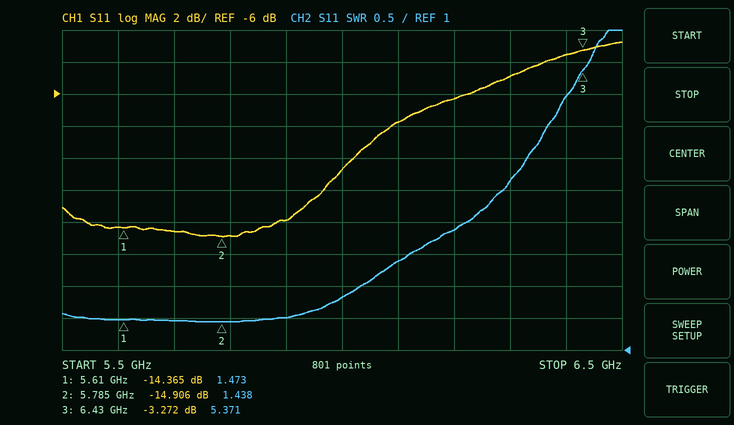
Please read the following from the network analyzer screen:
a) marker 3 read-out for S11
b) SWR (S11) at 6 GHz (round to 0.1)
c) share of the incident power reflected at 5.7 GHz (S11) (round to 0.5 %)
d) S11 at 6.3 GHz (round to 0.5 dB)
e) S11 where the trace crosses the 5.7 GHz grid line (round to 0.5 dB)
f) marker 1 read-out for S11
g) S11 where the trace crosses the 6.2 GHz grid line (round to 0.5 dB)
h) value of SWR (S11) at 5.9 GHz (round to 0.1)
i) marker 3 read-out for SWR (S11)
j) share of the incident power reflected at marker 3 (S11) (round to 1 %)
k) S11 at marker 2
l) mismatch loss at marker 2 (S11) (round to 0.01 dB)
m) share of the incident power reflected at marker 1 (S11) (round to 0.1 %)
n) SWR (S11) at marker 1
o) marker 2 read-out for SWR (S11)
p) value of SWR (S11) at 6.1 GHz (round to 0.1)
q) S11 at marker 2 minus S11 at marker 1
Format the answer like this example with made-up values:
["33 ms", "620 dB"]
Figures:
["-3.272 dB", "1.8", "3.5 %", "-5.0 dB", "-14.5 dB", "-14.365 dB", "-6.5 dB", "1.5", "5.371", "47 %", "-14.906 dB", "0.14 dB", "3.7 %", "1.473", "1.438", "2.4", "-0.541 dB"]
